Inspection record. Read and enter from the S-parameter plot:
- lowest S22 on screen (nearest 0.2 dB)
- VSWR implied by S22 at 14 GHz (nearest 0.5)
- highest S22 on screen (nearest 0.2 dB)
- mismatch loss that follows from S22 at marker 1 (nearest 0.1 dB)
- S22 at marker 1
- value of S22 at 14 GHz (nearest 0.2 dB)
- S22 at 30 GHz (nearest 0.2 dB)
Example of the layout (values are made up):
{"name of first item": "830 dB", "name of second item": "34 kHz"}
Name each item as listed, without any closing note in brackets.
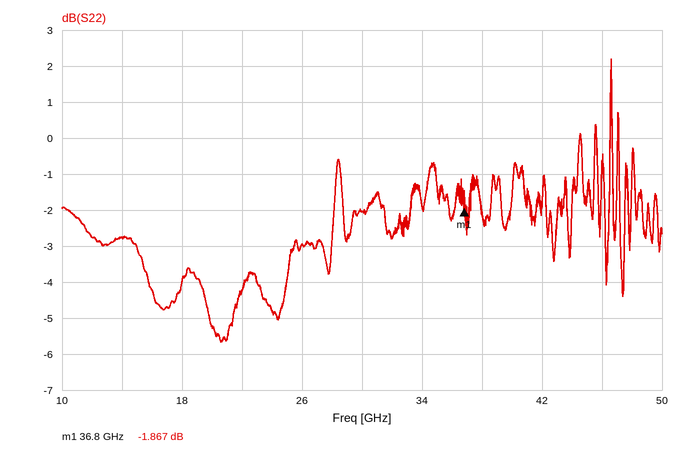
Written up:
{"lowest S22 on screen": "-5.6 dB", "VSWR implied by S22 at 14 GHz": "6.5", "highest S22 on screen": "2.2 dB", "mismatch loss that follows from S22 at marker 1": "4.6 dB", "S22 at marker 1": "-1.867 dB", "value of S22 at 14 GHz": "-2.8 dB", "S22 at 30 GHz": "-2.0 dB"}
